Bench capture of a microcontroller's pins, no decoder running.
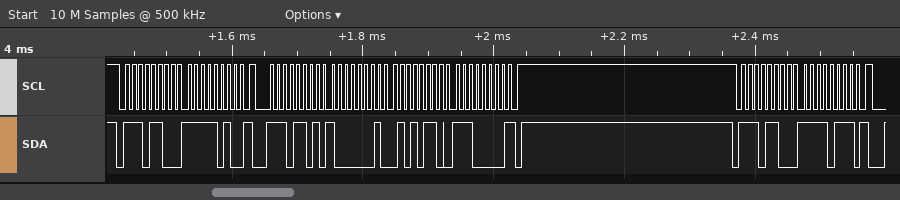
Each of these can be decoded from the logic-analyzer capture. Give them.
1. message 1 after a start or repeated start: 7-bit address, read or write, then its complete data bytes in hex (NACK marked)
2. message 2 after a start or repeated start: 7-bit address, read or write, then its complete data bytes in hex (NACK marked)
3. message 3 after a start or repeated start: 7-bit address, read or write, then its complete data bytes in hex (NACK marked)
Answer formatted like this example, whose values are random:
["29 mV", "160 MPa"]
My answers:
["0x76 write: FA", "0x76 read: 81 56 E0 NACK", "0x76 write: F7"]
